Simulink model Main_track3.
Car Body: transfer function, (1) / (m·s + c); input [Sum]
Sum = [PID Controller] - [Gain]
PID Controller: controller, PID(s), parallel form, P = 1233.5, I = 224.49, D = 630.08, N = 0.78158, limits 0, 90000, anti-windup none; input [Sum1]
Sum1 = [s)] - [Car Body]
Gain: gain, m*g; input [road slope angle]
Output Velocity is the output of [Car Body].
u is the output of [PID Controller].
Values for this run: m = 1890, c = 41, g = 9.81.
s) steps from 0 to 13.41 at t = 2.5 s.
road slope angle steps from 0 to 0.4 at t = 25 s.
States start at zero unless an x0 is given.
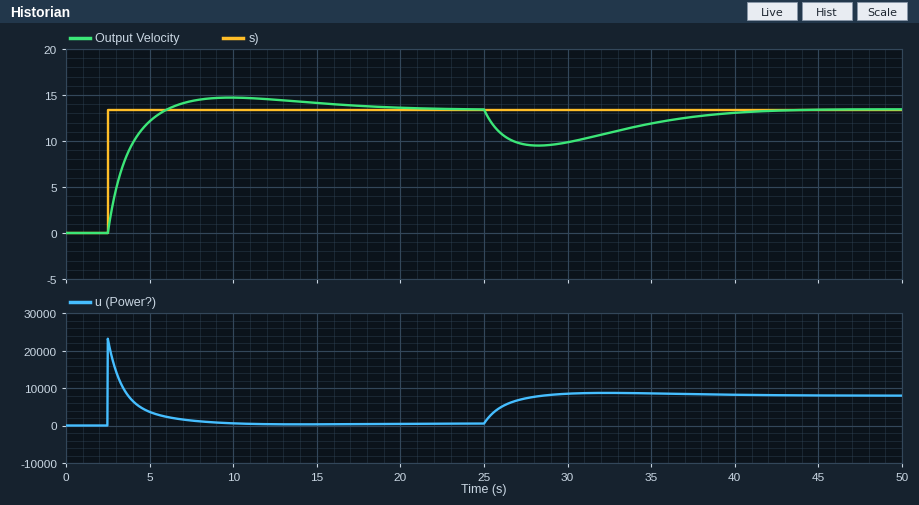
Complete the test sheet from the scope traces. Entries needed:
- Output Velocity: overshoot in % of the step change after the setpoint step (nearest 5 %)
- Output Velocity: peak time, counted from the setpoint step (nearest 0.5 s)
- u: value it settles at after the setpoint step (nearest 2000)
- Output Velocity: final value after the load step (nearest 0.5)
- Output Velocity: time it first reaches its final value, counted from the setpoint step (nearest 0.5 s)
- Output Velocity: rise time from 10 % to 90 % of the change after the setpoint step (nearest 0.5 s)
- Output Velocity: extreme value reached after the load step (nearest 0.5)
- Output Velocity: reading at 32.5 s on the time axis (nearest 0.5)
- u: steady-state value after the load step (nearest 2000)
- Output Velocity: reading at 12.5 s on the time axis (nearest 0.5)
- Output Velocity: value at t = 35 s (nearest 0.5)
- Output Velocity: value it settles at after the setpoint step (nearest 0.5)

10 %
7.5 s
0
13.5
3.5 s
2.5 s
9.5
11.0
8000
14.5
12.0
13.5
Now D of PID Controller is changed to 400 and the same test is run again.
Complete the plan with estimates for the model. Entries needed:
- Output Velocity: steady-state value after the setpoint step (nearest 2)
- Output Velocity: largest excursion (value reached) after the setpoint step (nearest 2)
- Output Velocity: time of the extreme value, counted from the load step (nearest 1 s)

14
14
3 s
